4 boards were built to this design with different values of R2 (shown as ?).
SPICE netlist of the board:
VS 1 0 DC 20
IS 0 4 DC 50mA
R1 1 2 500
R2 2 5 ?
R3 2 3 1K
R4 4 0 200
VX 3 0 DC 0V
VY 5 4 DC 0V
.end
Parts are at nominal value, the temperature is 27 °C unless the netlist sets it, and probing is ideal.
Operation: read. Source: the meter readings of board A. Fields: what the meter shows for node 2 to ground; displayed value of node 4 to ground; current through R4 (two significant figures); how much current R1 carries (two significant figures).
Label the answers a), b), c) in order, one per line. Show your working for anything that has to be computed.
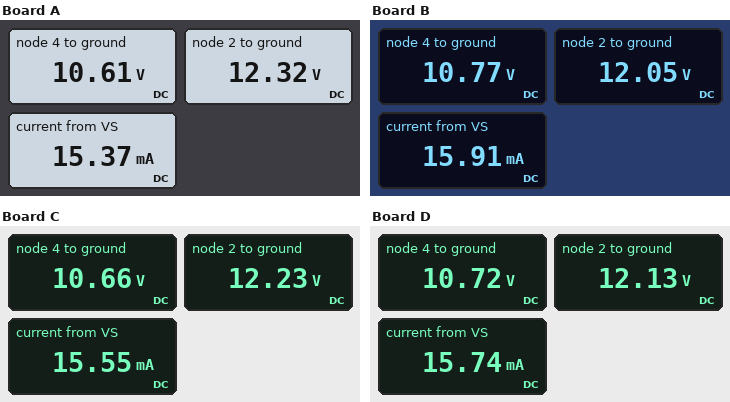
a) 12.32 V
b) 10.61 V
c) (10.61 V) / 200 Ω = 53 mA
d) (20 V - 12.32 V) / 500 Ω = 15 mA
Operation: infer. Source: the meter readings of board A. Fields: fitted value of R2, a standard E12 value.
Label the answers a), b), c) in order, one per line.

a) 560 Ω
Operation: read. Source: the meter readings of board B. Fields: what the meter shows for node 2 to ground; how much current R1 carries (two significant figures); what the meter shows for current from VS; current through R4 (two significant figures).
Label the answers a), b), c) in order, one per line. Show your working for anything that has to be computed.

a) 12.05 V
b) (20 V - 12.05 V) / 500 Ω = 16 mA
c) 15.91 mA
d) (10.77 V) / 200 Ω = 54 mA
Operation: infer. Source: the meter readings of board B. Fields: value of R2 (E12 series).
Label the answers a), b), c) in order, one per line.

a) 330 Ω
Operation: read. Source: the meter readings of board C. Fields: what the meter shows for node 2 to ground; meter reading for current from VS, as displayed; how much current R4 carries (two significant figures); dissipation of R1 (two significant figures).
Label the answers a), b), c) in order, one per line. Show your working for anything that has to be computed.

a) 12.23 V
b) 15.55 mA
c) (10.66 V) / 200 Ω = 53 mA
d) (20 V - 12.23 V)^2 / 500 Ω = 120 mW
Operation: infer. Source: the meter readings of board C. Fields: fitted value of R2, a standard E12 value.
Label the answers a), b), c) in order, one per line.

a) 470 Ω
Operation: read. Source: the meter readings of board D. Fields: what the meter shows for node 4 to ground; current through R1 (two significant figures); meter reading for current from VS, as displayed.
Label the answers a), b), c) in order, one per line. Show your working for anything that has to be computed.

a) 10.72 V
b) (20 V - 12.13 V) / 500 Ω = 16 mA
c) 15.74 mA
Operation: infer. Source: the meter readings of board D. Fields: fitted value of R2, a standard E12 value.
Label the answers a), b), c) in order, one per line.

a) 390 Ω
